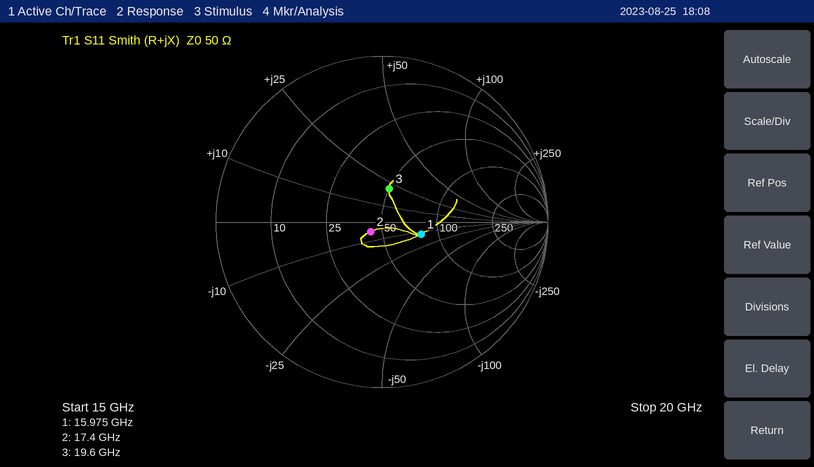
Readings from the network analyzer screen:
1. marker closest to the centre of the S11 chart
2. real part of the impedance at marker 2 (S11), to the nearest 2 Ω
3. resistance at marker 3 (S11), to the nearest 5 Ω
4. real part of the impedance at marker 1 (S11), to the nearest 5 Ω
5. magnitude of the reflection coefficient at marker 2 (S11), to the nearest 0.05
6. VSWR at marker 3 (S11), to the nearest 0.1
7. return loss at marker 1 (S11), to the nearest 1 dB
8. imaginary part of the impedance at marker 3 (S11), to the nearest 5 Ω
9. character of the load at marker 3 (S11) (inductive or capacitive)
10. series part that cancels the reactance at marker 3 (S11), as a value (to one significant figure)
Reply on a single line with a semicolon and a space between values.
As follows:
marker 2; 44 Ω; 50 Ω; 80 Ω; 0.10; 1.5; 12 dB; +20 Ω; inductive; 400 fF
